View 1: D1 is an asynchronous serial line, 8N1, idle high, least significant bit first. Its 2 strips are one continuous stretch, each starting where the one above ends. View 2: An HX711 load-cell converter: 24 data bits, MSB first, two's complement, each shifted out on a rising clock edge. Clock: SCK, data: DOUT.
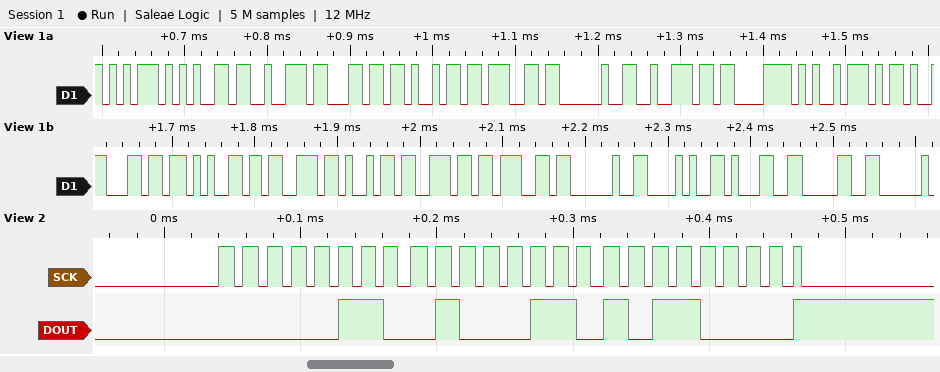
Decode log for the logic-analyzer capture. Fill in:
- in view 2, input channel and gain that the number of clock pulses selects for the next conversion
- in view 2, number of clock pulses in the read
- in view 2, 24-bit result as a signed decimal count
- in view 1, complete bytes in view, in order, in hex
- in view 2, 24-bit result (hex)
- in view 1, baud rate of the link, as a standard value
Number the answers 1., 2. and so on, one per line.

1. channel A, gain 128
2. 25
3. 411312
4. 0x75 0x65 0x72 0x6C 0x69 0x67 0x20 0x72 0xC3 0xA5 0x2D 0x6C 0x65 0x73 0x69 0x6E 0x67 0x20 0x28 0x31 0x30
5. 0x0646B0
6. 115200 baud
